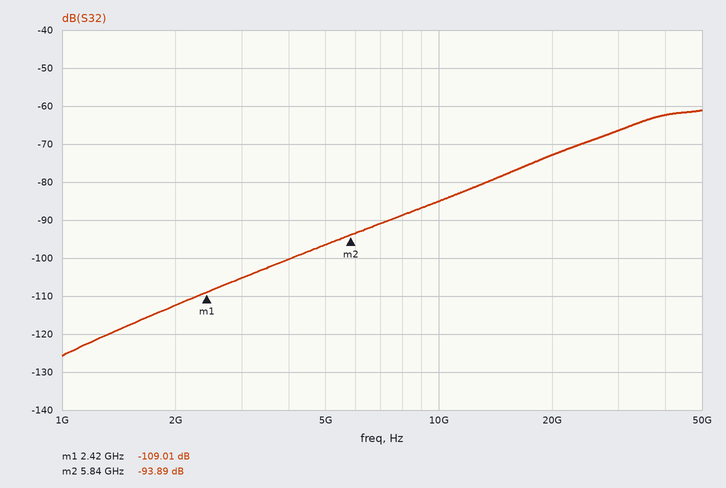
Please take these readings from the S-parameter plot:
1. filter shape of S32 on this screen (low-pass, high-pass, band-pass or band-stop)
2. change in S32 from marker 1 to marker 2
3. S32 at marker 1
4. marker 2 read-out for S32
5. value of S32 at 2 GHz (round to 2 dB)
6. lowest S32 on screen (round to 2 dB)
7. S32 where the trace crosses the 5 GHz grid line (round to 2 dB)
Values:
high-pass
15.12 dB
-109.01 dB
-93.89 dB
-112 dB
-126 dB
-96 dB
